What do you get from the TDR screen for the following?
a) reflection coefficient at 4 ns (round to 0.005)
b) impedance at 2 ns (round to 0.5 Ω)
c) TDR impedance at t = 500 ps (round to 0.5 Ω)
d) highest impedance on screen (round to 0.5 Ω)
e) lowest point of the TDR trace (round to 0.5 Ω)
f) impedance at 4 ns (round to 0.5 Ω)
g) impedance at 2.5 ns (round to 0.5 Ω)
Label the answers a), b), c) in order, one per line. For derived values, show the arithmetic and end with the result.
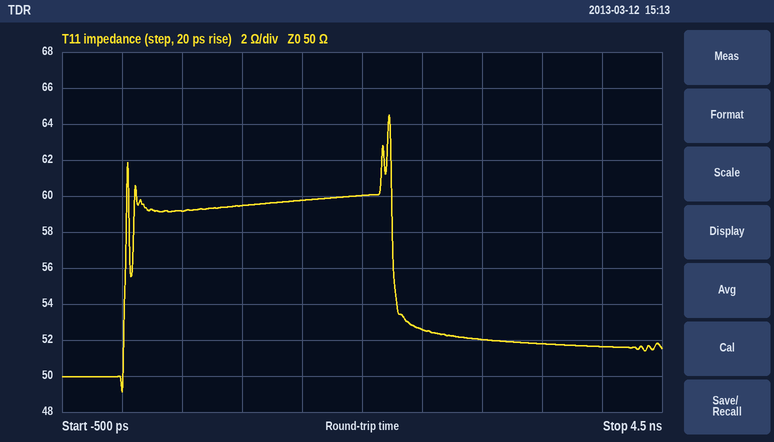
a) (51.5 − 50)/(51.5 + 50) ≈ +0.015
b) 60.0 Ω
c) 59.0 Ω
d) 64.5 Ω
e) 49.0 Ω
f) 51.5 Ω
g) 52.5 Ω
